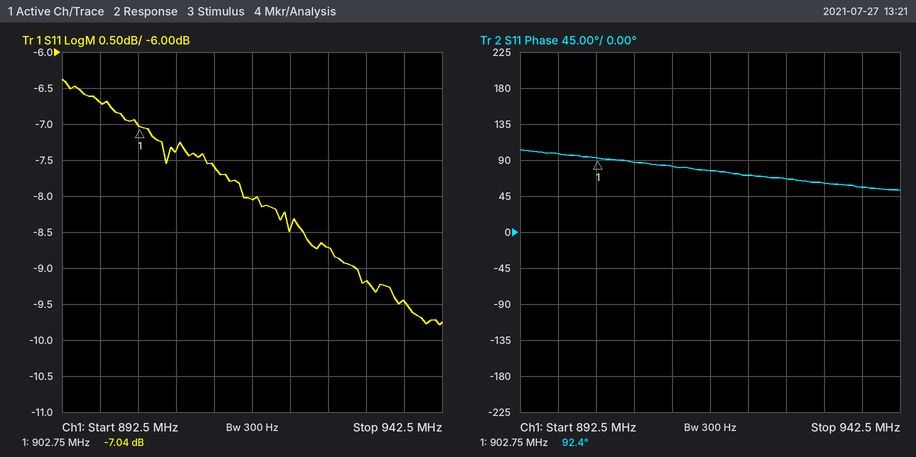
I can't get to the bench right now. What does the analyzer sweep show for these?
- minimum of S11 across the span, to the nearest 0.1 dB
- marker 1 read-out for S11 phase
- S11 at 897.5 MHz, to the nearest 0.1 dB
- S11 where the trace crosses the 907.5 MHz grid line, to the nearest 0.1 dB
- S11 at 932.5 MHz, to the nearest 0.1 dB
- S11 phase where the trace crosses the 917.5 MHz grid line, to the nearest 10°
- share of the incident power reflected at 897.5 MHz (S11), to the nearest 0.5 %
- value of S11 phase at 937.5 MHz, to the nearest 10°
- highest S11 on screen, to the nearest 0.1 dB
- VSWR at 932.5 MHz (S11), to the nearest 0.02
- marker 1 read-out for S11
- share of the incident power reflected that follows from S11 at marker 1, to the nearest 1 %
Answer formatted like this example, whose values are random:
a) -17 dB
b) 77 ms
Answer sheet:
a) -9.8 dB
b) 92.4°
c) -6.7 dB
d) -7.4 dB
e) -9.2 dB
f) 80°
g) 21.5 %
h) 60°
i) -6.4 dB
j) 2.06
k) -7.04 dB
l) 20 %
